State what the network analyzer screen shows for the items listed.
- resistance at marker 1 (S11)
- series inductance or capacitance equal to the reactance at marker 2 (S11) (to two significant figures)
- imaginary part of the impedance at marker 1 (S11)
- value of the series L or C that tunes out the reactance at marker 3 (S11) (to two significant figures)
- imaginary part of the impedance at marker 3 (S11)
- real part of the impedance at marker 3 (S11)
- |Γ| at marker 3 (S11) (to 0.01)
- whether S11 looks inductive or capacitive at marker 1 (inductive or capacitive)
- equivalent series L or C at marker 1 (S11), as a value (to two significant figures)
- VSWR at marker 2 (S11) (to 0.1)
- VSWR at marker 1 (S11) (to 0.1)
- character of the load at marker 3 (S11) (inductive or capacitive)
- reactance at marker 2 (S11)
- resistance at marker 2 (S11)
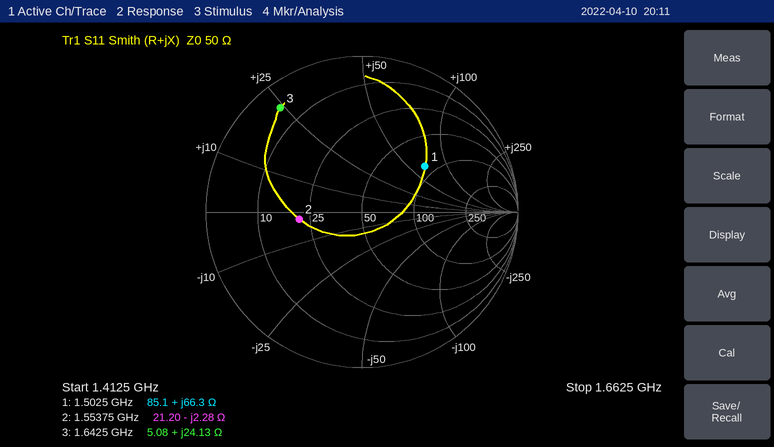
85.1 Ω
45 pF
+66.3 Ω
4.0 pF
+24.13 Ω
5.08 Ω
0.85
inductive
7.0 nH
2.4
3.0
inductive
-2.28 Ω
21.20 Ω
